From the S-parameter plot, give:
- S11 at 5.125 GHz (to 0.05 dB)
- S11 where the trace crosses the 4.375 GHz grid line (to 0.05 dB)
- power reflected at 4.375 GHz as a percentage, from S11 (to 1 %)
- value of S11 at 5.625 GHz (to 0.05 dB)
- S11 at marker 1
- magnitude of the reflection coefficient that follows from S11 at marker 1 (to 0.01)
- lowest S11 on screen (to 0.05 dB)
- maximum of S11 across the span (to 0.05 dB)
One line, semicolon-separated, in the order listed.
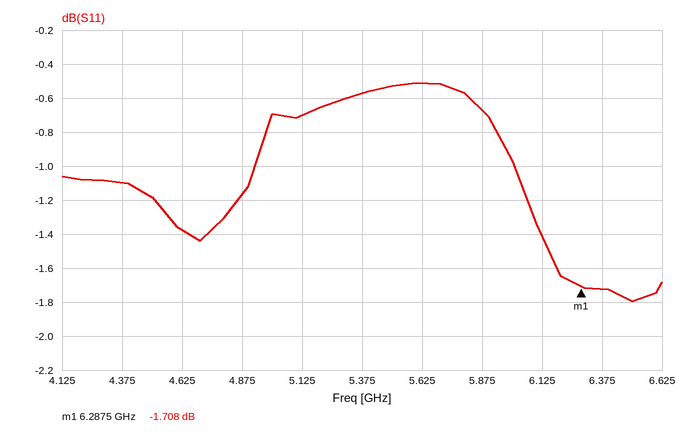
-0.70 dB; -1.10 dB; 78 %; -0.50 dB; -1.708 dB; 0.82; -1.80 dB; -0.50 dB
